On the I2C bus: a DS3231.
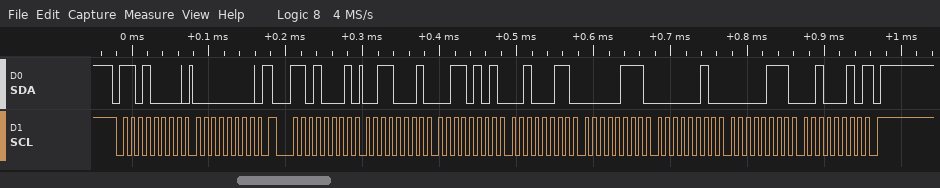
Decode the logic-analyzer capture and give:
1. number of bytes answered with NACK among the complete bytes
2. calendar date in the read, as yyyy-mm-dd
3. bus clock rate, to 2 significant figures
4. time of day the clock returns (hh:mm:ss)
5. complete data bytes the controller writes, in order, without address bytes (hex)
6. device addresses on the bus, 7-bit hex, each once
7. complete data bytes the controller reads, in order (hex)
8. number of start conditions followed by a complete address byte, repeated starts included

1
2022-07-02
100 kHz
23:35:31
00
0x68
31 35 23 07 02 07 22
2
